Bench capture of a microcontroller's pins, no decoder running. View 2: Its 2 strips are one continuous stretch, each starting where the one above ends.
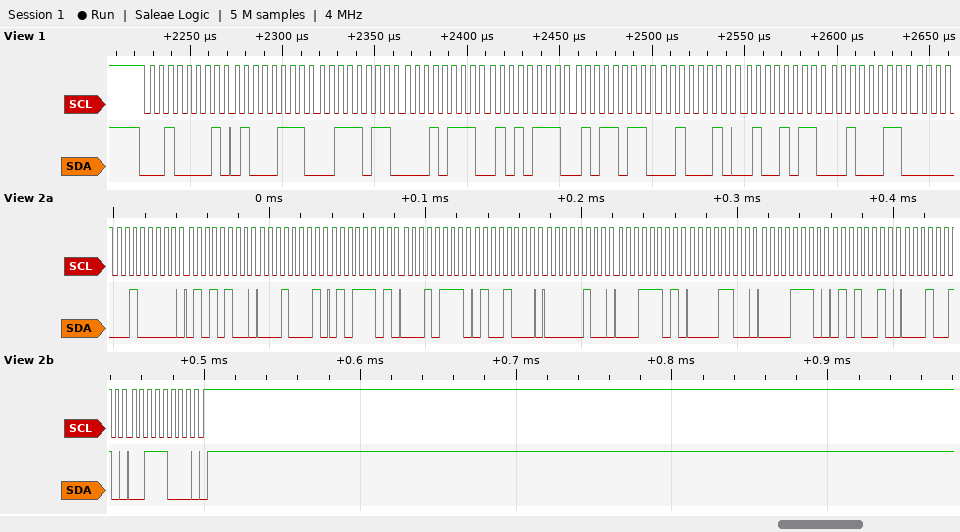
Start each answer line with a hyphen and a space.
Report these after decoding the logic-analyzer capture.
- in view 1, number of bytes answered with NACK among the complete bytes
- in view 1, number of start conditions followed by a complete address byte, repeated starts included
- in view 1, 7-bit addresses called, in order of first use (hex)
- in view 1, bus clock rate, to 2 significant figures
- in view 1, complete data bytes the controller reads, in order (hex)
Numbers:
- 0
- 1
- 0x10
- 200 kHz
- 47 3B 17 57 5B 22 4B 23
